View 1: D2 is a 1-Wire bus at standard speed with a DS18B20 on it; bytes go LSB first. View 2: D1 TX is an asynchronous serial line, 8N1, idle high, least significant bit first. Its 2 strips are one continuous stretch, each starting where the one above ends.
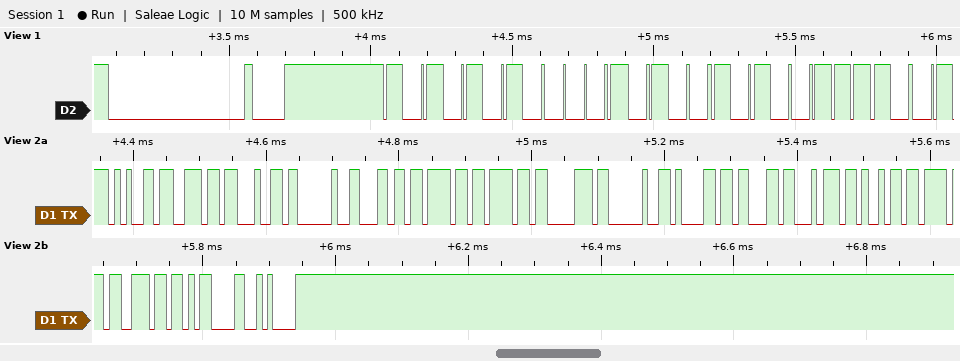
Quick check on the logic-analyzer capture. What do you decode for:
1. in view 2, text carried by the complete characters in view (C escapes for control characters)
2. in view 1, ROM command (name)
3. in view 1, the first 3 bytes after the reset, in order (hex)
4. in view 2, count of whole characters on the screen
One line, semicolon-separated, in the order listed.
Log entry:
"end loop action\r\n"; Match ROM; 55 28 E5; 17
